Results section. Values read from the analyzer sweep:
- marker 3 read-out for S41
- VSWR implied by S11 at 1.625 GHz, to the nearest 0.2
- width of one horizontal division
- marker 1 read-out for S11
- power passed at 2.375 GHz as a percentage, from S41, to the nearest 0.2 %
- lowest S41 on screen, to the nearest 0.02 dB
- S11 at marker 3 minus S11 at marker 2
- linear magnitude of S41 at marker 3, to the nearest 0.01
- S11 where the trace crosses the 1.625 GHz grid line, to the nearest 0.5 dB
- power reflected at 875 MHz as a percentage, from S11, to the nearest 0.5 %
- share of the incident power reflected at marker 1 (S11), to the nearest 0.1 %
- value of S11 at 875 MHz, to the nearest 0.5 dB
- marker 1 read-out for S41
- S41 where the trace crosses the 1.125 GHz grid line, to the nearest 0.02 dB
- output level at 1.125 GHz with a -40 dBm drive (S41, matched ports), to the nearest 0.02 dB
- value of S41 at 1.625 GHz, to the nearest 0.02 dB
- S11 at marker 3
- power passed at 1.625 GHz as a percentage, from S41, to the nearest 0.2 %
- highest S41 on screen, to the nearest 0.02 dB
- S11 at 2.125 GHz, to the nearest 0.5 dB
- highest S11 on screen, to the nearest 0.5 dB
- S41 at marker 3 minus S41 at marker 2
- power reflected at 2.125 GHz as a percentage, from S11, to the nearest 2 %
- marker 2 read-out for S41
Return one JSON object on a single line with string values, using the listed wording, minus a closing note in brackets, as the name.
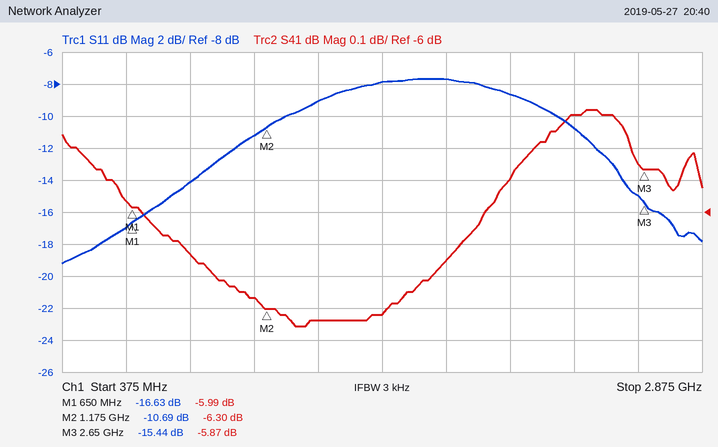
{"marker 3 read-out for S41": "-5.87 dB", "VSWR implied by S11 at 1.625 GHz, to the nearest 0.2": "2.4", "width of one horizontal division": "250 MHz", "marker 1 read-out for S11": "-16.63 dB", "power passed at 2.375 GHz as a percentage, from S41, to the nearest 0.2 %": "27.0 %", "lowest S41 on screen, to the nearest 0.02 dB": "-6.36 dB", "S11 at marker 3 minus S11 at marker 2": "-4.75 dB", "linear magnitude of S41 at marker 3, to the nearest 0.01": "0.51", "S11 where the trace crosses the 1.625 GHz grid line, to the nearest 0.5 dB": "-8.0 dB", "power reflected at 875 MHz as a percentage, from S11, to the nearest 0.5 %": "4.0 %", "share of the incident power reflected at marker 1 (S11), to the nearest 0.1 %": "2.2 %", "value of S11 at 875 MHz, to the nearest 0.5 dB": "-14.0 dB", "marker 1 read-out for S41": "-5.99 dB", "S41 where the trace crosses the 1.125 GHz grid line, to the nearest 0.02 dB": "-6.26 dB", "output level at 1.125 GHz with a -40 dBm drive (S41, matched ports), to the nearest 0.02 dB": "-46.26 dBm", "value of S41 at 1.625 GHz, to the nearest 0.02 dB": "-6.32 dB", "S11 at marker 3": "-15.44 dB", "power passed at 1.625 GHz as a percentage, from S41, to the nearest 0.2 %": "23.4 %", "highest S41 on screen, to the nearest 0.02 dB": "-5.68 dB", "S11 at 2.125 GHz, to the nearest 0.5 dB": "-8.5 dB", "highest S11 on screen, to the nearest 0.5 dB": "-7.5 dB", "S41 at marker 3 minus S41 at marker 2": "0.43 dB", "power reflected at 2.125 GHz as a percentage, from S11, to the nearest 2 %": "14 %", "marker 2 read-out for S41": "-6.30 dB"}
